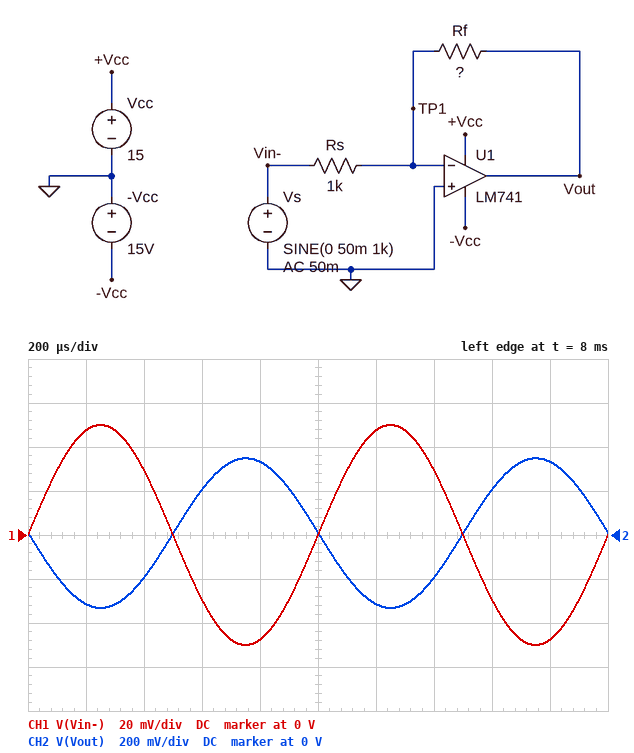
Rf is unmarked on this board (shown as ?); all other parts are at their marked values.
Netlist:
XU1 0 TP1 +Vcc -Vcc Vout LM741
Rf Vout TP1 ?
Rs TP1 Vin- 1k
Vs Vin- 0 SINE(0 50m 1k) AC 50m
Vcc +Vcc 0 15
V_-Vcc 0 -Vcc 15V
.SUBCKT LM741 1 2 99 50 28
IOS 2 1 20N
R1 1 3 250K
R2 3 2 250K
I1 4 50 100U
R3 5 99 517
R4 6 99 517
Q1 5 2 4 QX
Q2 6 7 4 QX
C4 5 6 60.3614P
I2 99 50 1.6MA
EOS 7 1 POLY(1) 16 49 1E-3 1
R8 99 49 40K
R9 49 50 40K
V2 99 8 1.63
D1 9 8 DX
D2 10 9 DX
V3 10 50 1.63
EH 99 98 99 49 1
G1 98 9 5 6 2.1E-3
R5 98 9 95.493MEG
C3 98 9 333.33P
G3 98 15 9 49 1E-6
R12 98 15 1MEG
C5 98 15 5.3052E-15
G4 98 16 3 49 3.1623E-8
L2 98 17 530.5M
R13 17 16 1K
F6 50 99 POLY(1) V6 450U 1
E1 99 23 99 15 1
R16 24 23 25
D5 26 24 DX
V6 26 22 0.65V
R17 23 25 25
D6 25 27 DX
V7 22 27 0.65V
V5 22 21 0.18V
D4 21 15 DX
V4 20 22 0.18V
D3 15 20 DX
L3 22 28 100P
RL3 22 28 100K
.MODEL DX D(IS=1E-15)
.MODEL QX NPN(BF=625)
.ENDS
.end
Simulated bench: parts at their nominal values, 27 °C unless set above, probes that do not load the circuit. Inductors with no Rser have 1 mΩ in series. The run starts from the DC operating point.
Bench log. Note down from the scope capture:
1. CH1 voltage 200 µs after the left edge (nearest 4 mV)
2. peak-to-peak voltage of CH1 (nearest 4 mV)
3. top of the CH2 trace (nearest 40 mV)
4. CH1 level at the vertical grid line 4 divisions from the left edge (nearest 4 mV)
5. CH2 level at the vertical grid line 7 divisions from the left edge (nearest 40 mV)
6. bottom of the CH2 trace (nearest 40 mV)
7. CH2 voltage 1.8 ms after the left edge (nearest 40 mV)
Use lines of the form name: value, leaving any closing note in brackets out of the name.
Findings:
CH1 voltage 200 µs after the left edge: 48 mV
peak-to-peak voltage of CH1: 100 mV
top of the CH2 trace: 360 mV
CH1 level at the vertical grid line 4 divisions from the left edge: -48 mV
CH2 level at the vertical grid line 7 divisions from the left edge: -200 mV
bottom of the CH2 trace: -320 mV
CH2 voltage 1.8 ms after the left edge: 320 mV
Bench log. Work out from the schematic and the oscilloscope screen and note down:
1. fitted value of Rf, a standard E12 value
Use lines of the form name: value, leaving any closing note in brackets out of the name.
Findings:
fitted value of Rf, a standard E12 value: 6.8 kΩ
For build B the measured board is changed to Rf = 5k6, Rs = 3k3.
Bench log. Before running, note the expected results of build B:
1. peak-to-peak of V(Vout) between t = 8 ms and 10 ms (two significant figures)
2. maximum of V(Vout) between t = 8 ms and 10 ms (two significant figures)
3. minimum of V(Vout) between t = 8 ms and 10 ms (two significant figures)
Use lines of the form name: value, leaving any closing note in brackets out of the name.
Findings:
peak-to-peak of V(Vout) between t = 8 ms and 10 ms: 170 mV
maximum of V(Vout) between t = 8 ms and 10 ms: 88 mV
minimum of V(Vout) between t = 8 ms and 10 ms: -82 mV
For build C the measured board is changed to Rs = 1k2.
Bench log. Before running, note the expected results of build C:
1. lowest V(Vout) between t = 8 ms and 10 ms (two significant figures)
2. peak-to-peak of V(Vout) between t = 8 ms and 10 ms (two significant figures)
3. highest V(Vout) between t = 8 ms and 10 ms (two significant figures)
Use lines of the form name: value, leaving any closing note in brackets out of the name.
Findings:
lowest V(Vout) between t = 8 ms and 10 ms: -280 mV
peak-to-peak of V(Vout) between t = 8 ms and 10 ms: 570 mV
highest V(Vout) between t = 8 ms and 10 ms: 290 mV
